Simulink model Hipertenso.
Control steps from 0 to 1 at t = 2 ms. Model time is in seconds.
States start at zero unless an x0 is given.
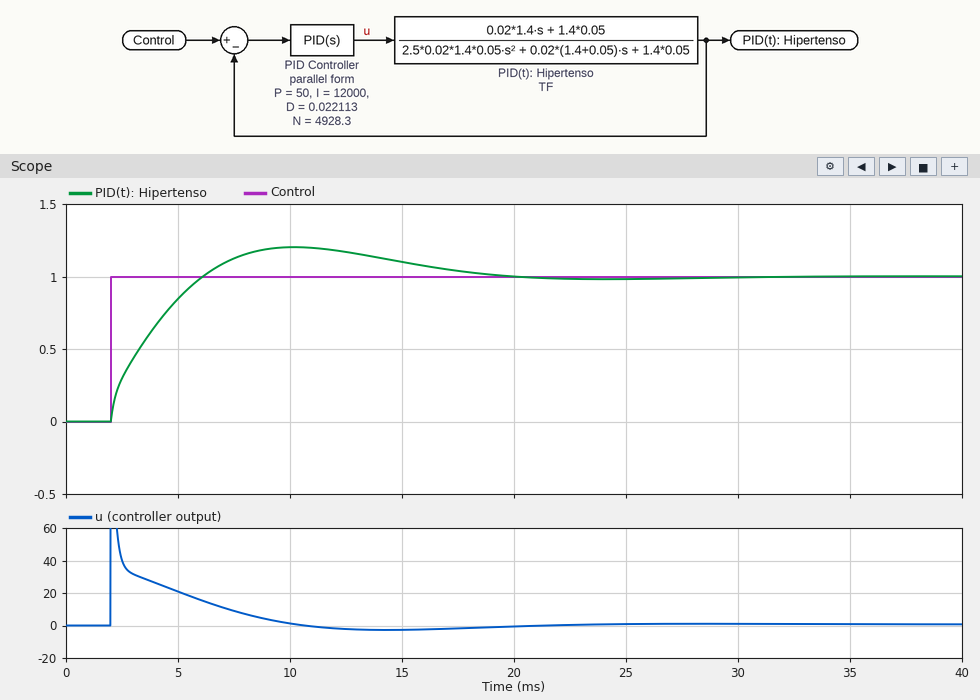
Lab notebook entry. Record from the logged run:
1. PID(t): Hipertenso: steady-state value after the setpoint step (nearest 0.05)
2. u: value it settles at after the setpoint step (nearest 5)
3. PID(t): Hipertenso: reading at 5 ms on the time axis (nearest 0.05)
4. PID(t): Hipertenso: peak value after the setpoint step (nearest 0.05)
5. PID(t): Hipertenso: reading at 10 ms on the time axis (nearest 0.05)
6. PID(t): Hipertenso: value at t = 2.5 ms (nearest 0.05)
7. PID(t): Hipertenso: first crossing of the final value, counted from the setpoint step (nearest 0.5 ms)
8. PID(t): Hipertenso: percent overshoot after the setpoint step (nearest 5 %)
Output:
1.00
0
0.85
1.20
1.20
0.30
4.0 ms
20 %
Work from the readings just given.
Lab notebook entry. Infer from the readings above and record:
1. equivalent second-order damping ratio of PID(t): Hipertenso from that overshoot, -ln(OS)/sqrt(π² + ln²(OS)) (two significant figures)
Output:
0.46
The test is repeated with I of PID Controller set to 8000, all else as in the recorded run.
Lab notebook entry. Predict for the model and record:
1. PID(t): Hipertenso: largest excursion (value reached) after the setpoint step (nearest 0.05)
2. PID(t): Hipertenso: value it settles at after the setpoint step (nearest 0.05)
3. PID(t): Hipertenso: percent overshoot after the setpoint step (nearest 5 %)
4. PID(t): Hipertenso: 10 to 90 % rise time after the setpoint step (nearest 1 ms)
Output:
1.15
1.00
15 %
4 ms
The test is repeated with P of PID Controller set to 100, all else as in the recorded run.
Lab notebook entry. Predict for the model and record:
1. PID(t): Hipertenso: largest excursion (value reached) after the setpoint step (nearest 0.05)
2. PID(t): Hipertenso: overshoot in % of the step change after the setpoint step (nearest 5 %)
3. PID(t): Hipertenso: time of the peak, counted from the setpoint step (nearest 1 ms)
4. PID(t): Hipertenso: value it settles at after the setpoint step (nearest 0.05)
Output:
1.10
10 %
7 ms
1.00
